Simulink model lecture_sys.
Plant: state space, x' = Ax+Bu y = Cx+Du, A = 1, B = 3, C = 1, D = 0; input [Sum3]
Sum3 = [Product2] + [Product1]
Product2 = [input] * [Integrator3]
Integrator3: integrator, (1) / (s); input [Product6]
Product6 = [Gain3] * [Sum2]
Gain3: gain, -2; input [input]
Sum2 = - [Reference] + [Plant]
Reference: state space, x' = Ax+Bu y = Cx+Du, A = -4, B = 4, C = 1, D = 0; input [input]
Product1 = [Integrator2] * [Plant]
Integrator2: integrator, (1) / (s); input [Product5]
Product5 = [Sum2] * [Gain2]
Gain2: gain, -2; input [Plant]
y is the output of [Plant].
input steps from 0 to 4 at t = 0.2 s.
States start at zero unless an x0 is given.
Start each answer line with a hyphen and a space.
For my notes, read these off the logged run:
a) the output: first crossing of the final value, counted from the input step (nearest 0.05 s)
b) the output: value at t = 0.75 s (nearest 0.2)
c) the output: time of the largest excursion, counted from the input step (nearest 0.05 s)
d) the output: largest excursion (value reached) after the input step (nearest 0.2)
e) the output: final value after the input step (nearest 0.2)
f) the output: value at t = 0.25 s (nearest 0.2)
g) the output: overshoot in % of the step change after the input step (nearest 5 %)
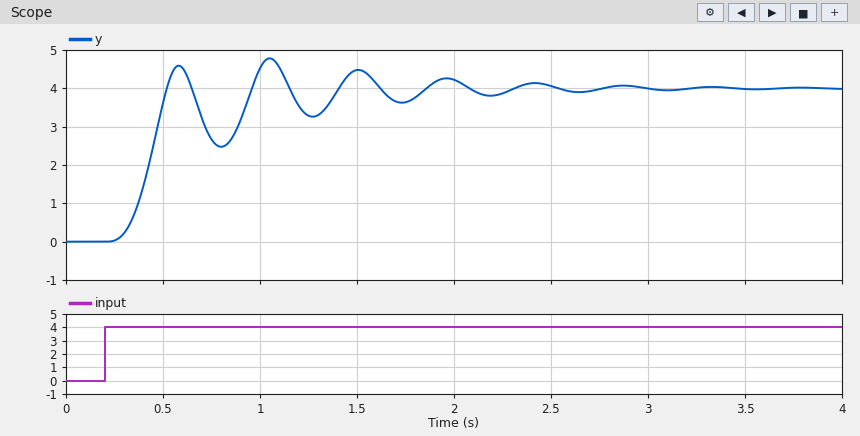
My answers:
- 0.30 s
- 2.6
- 0.85 s
- 4.8
- 4.0
- 0.0
- 20 %
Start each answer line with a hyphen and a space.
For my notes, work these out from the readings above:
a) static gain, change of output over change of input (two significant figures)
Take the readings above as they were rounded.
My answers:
- 1.0
